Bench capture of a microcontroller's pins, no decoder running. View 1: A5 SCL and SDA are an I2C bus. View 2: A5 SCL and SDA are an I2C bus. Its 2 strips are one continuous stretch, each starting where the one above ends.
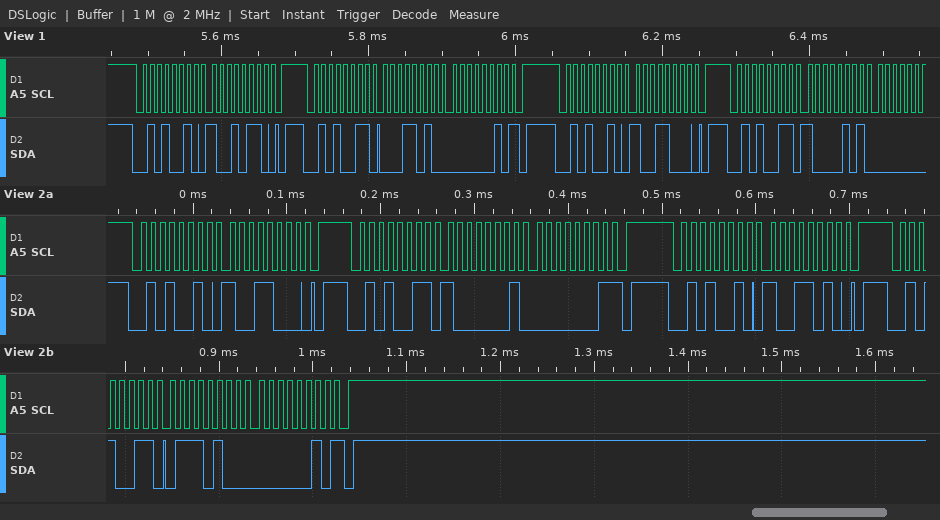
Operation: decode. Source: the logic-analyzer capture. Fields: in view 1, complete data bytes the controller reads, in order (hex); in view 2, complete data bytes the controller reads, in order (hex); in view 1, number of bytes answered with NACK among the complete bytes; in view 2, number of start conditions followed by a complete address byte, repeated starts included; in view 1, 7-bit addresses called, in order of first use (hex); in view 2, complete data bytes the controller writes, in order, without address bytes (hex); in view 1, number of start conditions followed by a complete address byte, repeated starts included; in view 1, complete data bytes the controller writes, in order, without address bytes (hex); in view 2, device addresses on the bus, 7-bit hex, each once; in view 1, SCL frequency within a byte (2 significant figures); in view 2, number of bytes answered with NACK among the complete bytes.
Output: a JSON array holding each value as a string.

["1A 02 85", "81 01 74 02", "1", "4", "0x29", "98 9A", "4", "96 98", "0x29", "100 kHz", "2"]
